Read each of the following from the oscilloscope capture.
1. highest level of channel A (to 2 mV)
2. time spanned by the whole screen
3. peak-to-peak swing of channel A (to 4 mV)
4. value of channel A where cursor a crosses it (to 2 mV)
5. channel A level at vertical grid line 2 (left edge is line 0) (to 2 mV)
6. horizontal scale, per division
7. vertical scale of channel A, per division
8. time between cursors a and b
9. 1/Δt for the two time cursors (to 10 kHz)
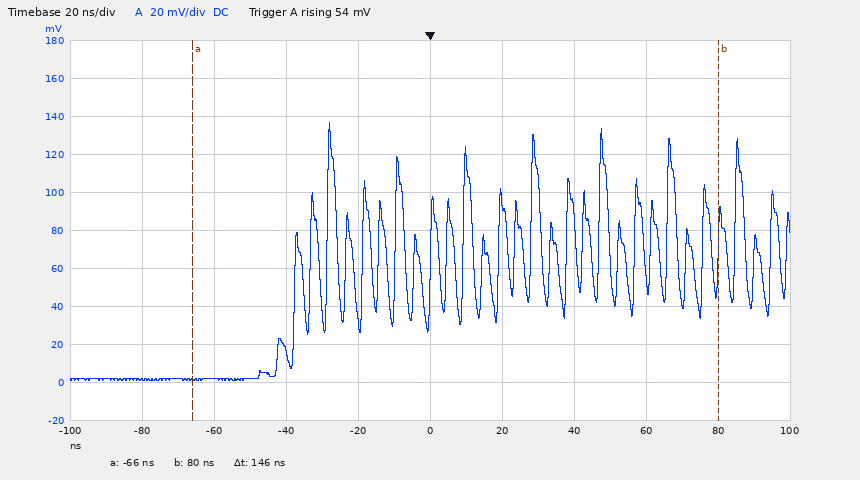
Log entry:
136 mV
200 ns
136 mV
2 mV
2 mV
20 ns
20 mV
146 ns
6.85 MHz
